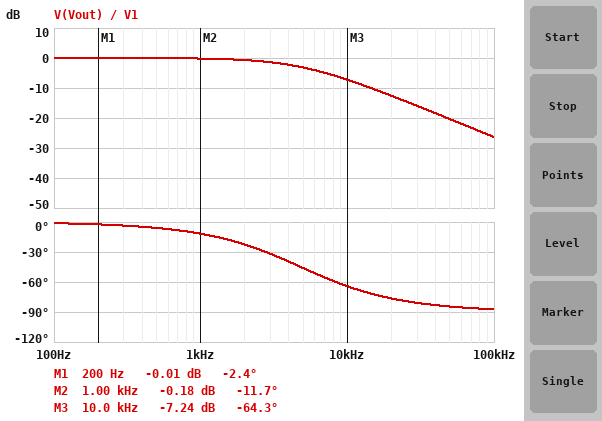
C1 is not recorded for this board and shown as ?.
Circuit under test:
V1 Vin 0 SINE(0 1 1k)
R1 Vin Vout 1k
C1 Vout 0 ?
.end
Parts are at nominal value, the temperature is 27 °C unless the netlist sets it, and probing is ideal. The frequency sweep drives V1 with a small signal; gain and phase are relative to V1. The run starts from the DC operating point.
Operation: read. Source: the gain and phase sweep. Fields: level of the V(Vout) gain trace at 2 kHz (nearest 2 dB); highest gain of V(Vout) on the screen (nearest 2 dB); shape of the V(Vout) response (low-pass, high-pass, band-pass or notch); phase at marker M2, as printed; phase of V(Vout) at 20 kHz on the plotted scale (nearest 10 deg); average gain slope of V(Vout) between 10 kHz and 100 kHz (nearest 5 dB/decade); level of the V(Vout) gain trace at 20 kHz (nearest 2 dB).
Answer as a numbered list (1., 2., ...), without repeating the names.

1. 0 dB
2. 0 dB
3. low-pass
4. -11.7 deg
5. -80 deg
6. -20 dB/decade
7. -12 dB
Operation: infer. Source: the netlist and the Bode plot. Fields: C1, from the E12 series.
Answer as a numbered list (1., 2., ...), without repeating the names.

1. 33 nF
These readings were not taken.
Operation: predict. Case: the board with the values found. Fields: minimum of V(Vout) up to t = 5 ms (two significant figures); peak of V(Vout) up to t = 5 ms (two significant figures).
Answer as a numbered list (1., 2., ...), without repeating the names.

1. -980 mV
2. 980 mV
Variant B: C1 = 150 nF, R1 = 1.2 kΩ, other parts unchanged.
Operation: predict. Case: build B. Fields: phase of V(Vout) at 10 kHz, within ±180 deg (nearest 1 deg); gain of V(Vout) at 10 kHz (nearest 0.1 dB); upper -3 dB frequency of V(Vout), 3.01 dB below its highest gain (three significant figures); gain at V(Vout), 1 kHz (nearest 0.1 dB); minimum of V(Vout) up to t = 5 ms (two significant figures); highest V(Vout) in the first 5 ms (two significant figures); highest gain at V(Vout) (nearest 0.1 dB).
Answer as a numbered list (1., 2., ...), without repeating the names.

1. -85 deg
2. -21.1 dB
3. 884 Hz
4. -3.6 dB
5. -660 mV
6. 720 mV
7. 0 dB
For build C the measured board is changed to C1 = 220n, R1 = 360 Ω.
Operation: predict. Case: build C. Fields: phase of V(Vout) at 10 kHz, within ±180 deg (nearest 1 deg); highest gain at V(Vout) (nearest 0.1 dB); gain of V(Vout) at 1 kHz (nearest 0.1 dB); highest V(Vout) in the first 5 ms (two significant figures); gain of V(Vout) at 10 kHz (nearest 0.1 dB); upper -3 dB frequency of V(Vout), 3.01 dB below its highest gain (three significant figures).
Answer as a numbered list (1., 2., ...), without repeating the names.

1. -79 deg
2. 0 dB
3. -1.0 dB
4. 900 mV
5. -14.1 dB
6. 2.01 kHz
